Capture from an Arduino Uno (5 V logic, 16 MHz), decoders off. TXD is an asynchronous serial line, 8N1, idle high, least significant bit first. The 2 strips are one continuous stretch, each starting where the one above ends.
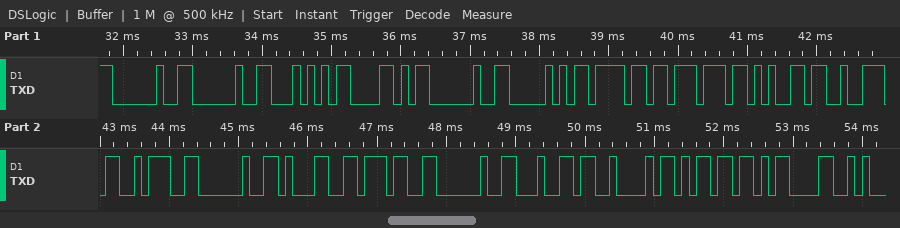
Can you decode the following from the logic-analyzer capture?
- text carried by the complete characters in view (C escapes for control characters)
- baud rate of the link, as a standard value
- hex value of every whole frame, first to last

"  TX Power: 17 dBm\r"
9600 baud
20 20 54 58 20 50 6F 77 65 72 3A 20 31 37 20 64 42 6D 0D
